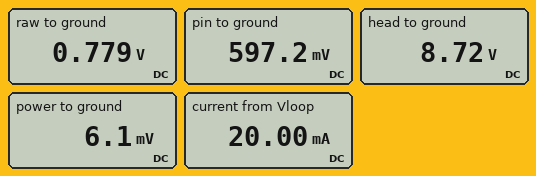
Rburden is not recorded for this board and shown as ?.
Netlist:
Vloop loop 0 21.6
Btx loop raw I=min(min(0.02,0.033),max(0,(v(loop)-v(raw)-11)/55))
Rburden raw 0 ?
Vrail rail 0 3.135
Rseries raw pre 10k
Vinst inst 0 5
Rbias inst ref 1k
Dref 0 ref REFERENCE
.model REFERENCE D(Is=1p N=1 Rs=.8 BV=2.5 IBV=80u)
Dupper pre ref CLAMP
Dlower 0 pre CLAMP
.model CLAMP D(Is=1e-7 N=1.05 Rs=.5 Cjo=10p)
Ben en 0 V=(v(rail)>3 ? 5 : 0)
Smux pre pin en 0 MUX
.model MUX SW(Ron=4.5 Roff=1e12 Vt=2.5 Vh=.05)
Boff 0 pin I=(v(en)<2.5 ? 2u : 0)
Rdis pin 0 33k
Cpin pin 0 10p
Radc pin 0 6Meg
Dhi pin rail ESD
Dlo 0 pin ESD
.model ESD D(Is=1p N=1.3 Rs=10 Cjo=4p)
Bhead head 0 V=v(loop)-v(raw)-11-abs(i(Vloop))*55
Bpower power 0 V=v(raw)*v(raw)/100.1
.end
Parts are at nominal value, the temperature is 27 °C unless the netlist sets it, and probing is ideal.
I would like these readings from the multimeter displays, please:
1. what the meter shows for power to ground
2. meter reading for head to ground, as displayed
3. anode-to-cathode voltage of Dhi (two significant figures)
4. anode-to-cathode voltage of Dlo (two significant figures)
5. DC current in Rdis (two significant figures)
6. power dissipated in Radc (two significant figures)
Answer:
6.1 mV
8.72 V
-2.5 V
-600 mV
18 µA
59 nW
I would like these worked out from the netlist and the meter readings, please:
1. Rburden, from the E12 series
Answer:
39 Ω
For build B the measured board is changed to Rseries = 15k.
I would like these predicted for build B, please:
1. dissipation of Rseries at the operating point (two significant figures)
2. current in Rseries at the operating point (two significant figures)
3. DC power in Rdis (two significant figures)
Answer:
4.0 µW
16 µA
8.7 µW
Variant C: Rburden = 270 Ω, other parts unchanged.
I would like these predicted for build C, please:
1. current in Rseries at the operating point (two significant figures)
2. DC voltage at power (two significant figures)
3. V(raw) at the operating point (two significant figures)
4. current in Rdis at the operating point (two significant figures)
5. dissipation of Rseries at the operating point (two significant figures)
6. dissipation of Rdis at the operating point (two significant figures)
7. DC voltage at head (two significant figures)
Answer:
250 µA
280 mV
5.3 V
85 µA
640 µW
240 µW
4.2 V
